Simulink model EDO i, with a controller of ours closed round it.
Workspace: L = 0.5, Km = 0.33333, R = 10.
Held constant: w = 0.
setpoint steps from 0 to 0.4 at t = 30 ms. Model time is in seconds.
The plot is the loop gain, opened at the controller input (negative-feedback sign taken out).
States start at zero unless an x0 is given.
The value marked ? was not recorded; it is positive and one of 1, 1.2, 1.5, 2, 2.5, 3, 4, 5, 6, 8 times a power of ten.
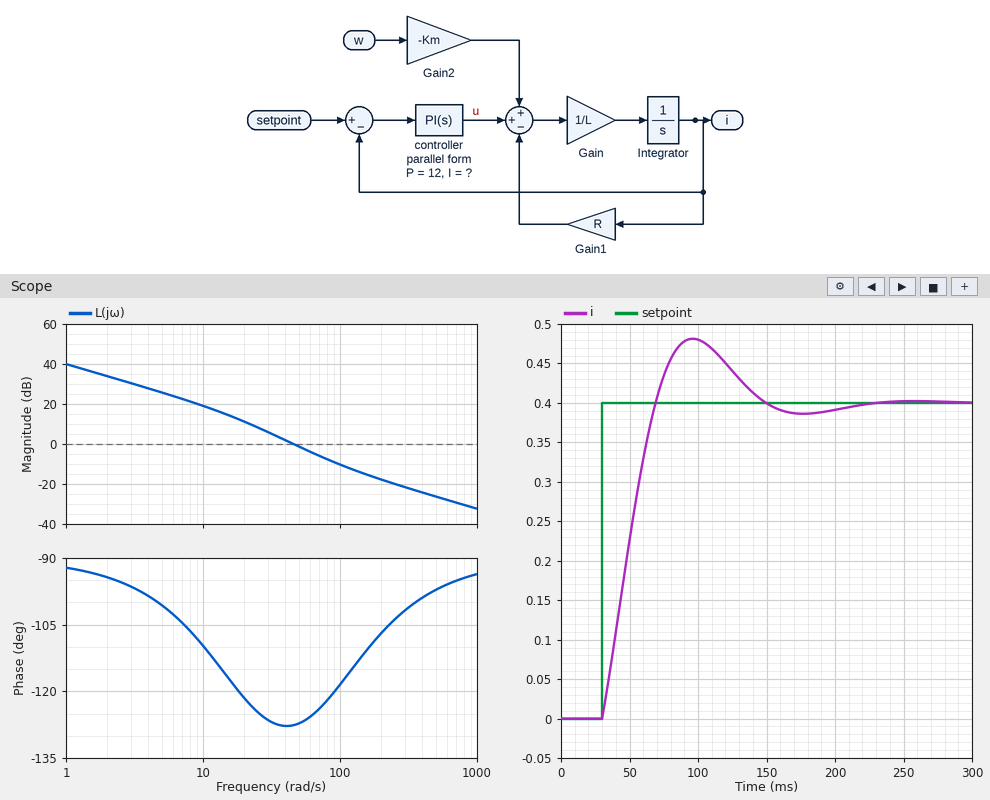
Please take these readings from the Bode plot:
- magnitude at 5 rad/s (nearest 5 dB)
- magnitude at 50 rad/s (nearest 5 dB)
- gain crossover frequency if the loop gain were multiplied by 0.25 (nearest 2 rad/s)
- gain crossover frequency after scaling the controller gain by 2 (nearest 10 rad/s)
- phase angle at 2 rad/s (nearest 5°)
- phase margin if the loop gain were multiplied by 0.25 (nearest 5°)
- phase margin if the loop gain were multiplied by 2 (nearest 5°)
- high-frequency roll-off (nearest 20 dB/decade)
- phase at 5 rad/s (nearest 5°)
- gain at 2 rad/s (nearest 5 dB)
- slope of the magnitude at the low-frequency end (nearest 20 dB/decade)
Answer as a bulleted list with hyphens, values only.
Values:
- 25 dB
- 0 dB
- 18 rad/s
- 70 rad/s
- -95°
- 60°
- 55°
- -20 dB/decade
- -100°
- 35 dB
- -20 dB/decade
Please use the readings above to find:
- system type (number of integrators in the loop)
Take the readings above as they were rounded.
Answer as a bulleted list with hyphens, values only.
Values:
- 1
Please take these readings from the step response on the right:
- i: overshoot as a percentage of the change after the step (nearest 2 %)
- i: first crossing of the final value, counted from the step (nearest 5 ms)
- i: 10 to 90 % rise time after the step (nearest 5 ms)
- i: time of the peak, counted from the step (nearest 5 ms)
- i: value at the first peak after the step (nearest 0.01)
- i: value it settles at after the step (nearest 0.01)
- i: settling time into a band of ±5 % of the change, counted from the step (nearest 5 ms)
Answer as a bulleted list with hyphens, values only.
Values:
- 20 %
- 40 ms
- 30 ms
- 65 ms
- 0.48
- 0.40
- 105 ms
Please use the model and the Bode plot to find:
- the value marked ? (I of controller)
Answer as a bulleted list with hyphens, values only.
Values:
- 1000
